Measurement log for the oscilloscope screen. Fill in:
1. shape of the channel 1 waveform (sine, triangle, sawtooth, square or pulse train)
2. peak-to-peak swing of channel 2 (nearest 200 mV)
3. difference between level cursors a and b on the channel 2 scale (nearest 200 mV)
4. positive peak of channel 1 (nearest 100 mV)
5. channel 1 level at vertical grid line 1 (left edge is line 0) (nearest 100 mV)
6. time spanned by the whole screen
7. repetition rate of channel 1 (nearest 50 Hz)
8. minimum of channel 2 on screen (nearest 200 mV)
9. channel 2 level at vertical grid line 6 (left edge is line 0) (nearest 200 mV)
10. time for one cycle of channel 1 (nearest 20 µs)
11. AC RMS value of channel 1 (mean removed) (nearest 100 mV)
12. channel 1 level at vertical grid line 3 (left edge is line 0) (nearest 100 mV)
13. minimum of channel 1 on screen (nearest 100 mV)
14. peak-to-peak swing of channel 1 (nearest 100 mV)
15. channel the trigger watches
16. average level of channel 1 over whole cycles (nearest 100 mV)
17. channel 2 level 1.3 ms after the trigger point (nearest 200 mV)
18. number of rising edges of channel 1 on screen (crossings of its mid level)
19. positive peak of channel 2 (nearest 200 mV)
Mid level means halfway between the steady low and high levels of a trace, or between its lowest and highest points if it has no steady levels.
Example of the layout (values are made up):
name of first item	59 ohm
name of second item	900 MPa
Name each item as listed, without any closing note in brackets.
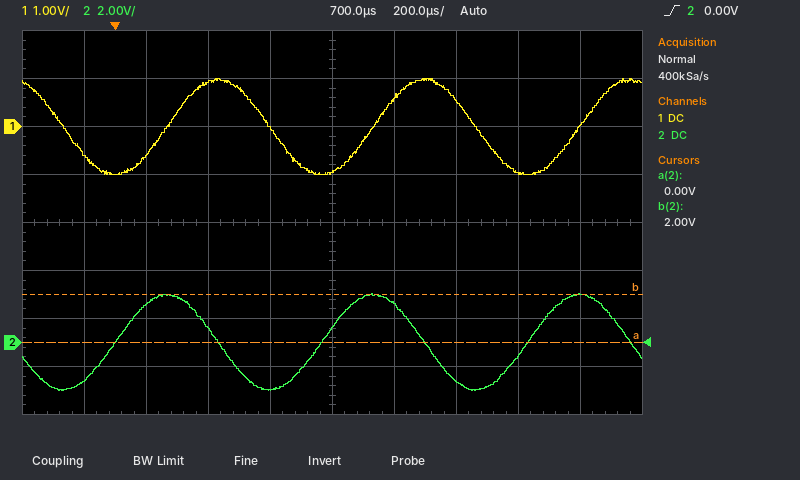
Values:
shape of the channel 1 waveform	sine
peak-to-peak swing of channel 2	4.0 V
difference between level cursors a and b on the channel 2 scale	2.0 V
positive peak of channel 1	1.0 V
channel 1 level at vertical grid line 1 (left edge is line 0)	-600 mV
time spanned by the whole screen	2 ms
repetition rate of channel 1	1.50 kHz
minimum of channel 2 on screen	-2.0 V
channel 2 level at vertical grid line 6 (left edge is line 0)	1.6 V
time for one cycle of channel 1	660 µs
AC RMS value of channel 1 (mean removed)	700 mV
channel 1 level at vertical grid line 3 (left edge is line 0)	900 mV
minimum of channel 1 on screen	-1.0 V
peak-to-peak swing of channel 1	2.0 V
channel the trigger watches	channel 2
average level of channel 1 over whole cycles	0.0 V
channel 2 level 1.3 ms after the trigger point	-600 mV
number of rising edges of channel 1 on screen	3
positive peak of channel 2	2.0 V
